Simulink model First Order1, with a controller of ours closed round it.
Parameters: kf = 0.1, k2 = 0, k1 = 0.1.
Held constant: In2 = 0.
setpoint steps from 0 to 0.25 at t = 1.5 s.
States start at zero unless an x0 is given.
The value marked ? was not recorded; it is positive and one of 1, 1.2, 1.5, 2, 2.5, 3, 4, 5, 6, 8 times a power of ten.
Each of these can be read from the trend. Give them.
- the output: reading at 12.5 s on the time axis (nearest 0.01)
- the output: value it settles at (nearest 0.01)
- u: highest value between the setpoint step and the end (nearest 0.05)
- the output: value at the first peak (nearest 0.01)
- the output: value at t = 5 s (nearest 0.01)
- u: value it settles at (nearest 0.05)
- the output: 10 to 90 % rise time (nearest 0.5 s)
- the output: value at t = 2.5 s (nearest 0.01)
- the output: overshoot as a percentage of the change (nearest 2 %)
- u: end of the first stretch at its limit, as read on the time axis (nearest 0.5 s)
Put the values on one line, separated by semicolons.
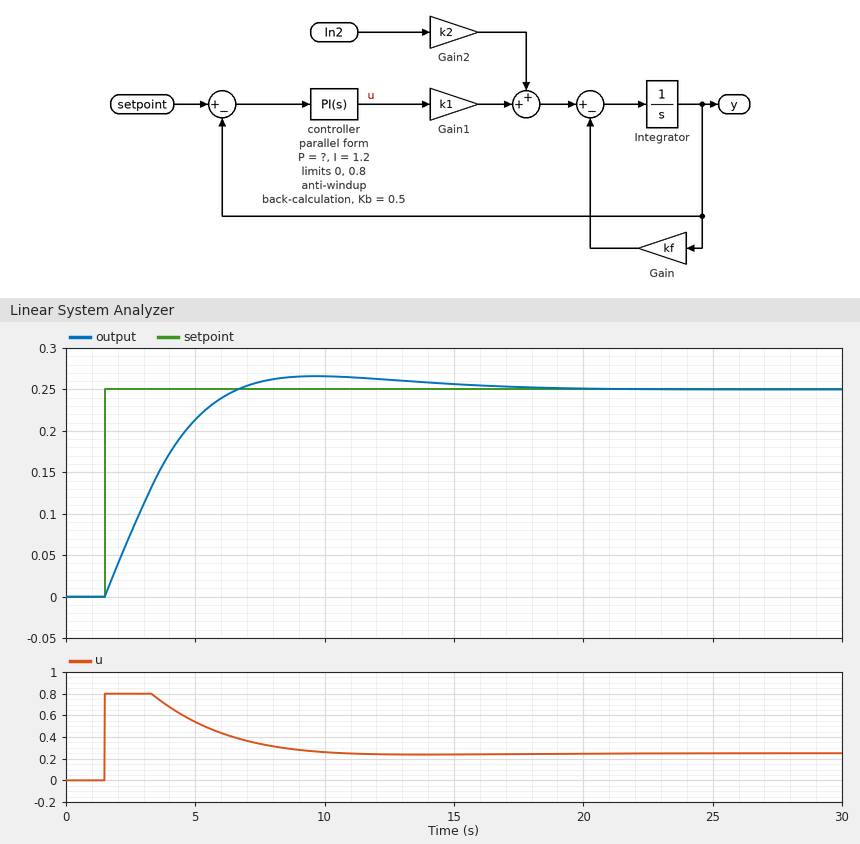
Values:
0.26; 0.25; 0.80; 0.27; 0.21; 0.25; 3.5 s; 0.08; 6 %; 3.5 s
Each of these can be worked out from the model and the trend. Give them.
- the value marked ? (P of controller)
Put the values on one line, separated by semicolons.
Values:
5
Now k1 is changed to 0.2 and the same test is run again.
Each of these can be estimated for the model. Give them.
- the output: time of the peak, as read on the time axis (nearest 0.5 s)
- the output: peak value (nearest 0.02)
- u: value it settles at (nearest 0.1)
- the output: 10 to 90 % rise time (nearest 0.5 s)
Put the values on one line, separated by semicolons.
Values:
6.5 s; 0.26; 0.1; 2.0 s
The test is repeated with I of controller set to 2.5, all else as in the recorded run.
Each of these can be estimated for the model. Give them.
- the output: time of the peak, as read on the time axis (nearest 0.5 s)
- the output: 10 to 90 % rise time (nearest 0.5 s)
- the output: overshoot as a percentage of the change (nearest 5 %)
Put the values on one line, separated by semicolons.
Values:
7.5 s; 3.0 s; 15 %
